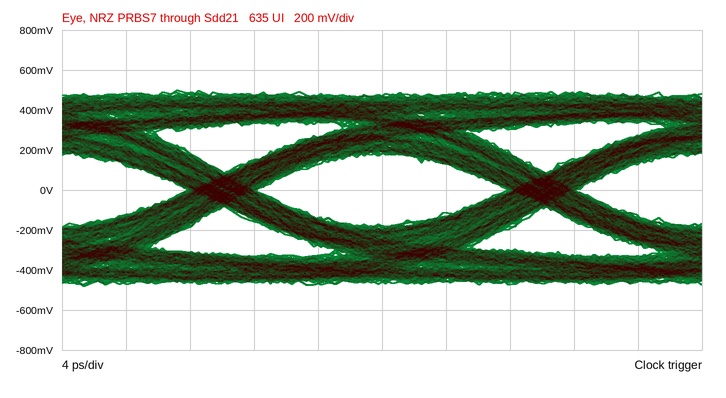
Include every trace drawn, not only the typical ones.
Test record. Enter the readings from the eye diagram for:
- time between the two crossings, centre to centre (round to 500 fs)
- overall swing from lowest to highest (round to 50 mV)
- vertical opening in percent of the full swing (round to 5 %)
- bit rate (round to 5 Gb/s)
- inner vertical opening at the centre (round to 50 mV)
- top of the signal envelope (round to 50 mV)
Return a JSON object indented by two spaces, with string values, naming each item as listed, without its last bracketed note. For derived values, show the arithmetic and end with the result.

{
  "time between the two crossings, centre to centre": "20.0 ps",
  "overall swing from lowest to highest": "1.00 V",
  "vertical opening in percent of the full swing": "350 mV / 1.00 V ≈ 35 %",
  "bit rate": "50 Gb/s",
  "inner vertical opening at the centre": "350 mV",
  "top of the signal envelope": "500 mV"
}
